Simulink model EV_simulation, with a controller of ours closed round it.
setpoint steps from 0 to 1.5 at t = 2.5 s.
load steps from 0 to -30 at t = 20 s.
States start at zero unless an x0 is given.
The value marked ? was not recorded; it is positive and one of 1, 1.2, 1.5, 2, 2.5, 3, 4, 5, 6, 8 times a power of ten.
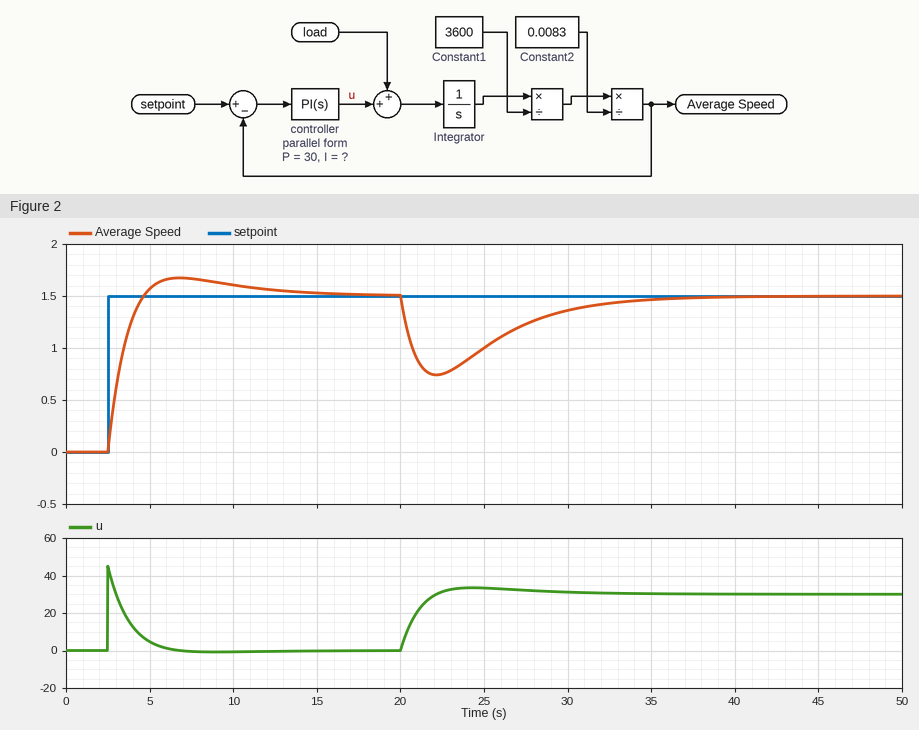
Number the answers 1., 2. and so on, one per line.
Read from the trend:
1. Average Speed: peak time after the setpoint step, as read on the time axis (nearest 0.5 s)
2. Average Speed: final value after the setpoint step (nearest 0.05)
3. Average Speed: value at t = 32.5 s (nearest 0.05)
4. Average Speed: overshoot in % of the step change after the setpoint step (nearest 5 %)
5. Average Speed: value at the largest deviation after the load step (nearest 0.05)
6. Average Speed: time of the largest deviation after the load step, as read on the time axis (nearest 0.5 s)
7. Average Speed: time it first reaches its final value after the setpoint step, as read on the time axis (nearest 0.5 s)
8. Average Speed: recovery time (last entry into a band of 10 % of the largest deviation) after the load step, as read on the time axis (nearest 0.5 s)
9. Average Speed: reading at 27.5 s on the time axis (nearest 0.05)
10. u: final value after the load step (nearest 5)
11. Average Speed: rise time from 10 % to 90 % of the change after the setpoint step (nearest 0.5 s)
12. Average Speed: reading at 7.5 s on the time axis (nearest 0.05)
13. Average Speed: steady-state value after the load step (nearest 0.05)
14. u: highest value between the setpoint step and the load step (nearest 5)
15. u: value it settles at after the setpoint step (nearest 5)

1. 7.0 s
2. 1.50
3. 1.45
4. 10 %
5. 0.75
6. 22.0 s
7. 4.5 s
8. 32.0 s
9. 1.25
10. 30
11. 1.5 s
12. 1.65
13. 1.50
14. 45
15. 0
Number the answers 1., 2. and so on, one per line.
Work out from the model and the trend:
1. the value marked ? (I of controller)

1. 6
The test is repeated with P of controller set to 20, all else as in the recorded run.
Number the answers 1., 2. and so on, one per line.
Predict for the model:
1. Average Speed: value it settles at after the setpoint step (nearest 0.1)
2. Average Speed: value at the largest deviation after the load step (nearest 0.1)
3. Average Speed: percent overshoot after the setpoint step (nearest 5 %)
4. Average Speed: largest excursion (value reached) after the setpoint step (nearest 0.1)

1. 1.5
2. 0.5
3. 20 %
4. 1.8
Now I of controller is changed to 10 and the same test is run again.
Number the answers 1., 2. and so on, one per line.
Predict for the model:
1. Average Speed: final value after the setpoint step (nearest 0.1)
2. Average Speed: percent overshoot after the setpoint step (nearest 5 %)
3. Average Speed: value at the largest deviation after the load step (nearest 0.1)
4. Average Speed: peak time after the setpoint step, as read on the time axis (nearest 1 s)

1. 1.5
2. 15 %
3. 0.8
4. 6 s
